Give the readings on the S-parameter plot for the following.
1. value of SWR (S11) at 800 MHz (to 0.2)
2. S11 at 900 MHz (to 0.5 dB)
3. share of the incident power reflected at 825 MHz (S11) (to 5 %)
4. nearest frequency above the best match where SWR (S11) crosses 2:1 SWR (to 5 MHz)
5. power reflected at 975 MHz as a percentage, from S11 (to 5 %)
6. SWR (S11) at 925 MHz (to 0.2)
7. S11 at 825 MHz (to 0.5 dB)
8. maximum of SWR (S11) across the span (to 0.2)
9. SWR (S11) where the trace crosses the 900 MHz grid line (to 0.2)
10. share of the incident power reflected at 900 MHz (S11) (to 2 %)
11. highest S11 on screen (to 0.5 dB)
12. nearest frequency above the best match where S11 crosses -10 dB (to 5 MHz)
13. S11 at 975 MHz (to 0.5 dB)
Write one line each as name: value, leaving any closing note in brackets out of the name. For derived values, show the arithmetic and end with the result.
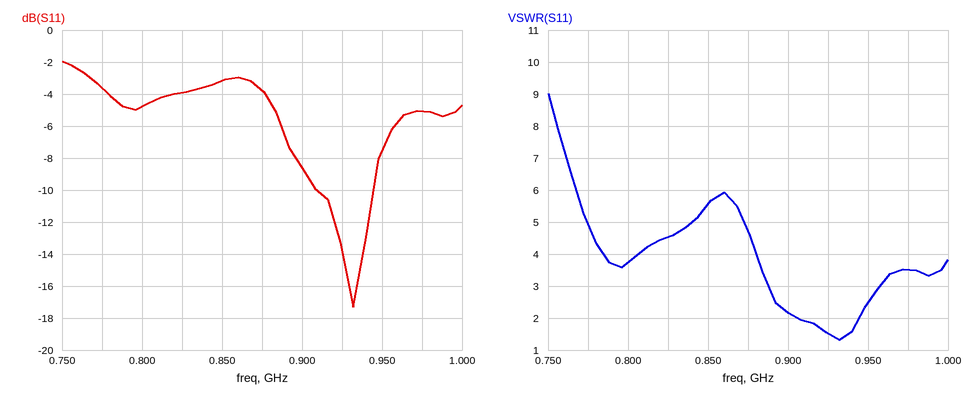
value of SWR (S11) at 800 MHz: 3.8
S11 at 900 MHz: -8.5 dB
share of the incident power reflected at 825 MHz (S11): 10^(-4/10) ≈ 40 %
nearest frequency above the best match where SWR (S11) crosses 2:1 SWR: 945 MHz
power reflected at 975 MHz as a percentage, from S11: 10^(-5/10) ≈ 31.6 %, so 30 % to the nearest 5 %
SWR (S11) at 925 MHz: 1.6
S11 at 825 MHz: -4.0 dB
maximum of SWR (S11) across the span: 9.0
SWR (S11) where the trace crosses the 900 MHz grid line: 2.2
share of the incident power reflected at 900 MHz (S11): 10^(-8.5/10) ≈ 14 %
highest S11 on screen: -2.0 dB
nearest frequency above the best match where S11 crosses -10 dB: 945 MHz
S11 at 975 MHz: -5.0 dB
